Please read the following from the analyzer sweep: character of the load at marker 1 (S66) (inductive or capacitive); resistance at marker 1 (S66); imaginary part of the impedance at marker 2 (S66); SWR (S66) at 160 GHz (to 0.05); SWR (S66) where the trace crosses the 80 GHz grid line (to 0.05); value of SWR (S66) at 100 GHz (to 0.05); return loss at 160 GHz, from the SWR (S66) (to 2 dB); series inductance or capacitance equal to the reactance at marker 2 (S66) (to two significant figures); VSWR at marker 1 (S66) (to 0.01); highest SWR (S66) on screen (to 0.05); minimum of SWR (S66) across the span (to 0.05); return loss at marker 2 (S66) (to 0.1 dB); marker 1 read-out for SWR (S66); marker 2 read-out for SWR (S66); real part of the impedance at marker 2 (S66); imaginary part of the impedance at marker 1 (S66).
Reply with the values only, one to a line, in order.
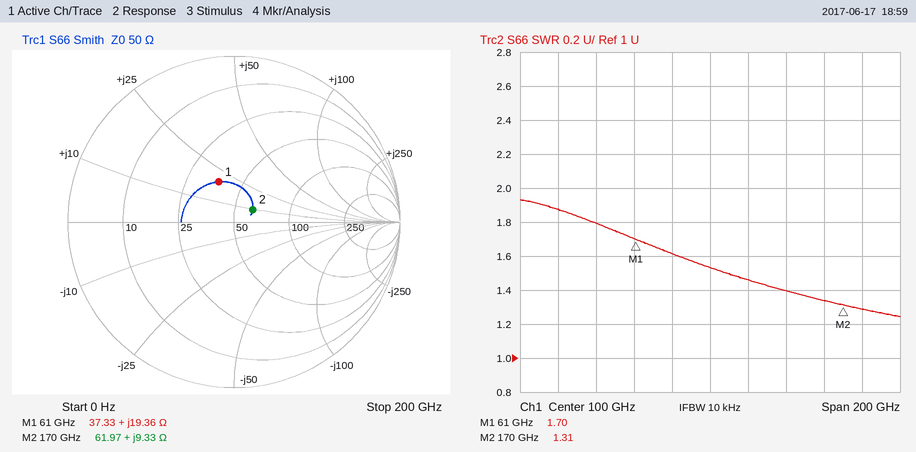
inductive
37.33 Ω
+9.33 Ω
1.35
1.60
1.55
16 dB
8.7 pH
1.70
1.95
1.25
17.4 dB
1.70
1.31
61.97 Ω
+19.36 Ω
